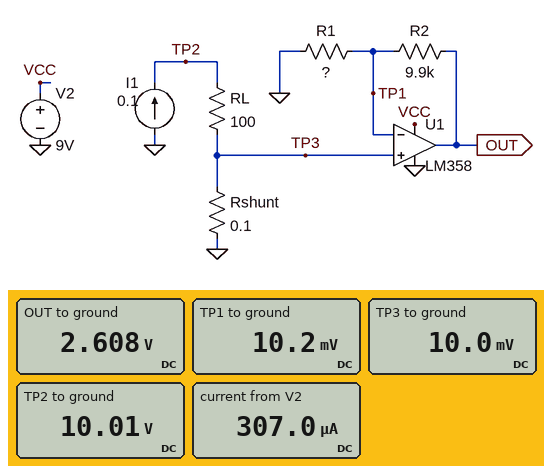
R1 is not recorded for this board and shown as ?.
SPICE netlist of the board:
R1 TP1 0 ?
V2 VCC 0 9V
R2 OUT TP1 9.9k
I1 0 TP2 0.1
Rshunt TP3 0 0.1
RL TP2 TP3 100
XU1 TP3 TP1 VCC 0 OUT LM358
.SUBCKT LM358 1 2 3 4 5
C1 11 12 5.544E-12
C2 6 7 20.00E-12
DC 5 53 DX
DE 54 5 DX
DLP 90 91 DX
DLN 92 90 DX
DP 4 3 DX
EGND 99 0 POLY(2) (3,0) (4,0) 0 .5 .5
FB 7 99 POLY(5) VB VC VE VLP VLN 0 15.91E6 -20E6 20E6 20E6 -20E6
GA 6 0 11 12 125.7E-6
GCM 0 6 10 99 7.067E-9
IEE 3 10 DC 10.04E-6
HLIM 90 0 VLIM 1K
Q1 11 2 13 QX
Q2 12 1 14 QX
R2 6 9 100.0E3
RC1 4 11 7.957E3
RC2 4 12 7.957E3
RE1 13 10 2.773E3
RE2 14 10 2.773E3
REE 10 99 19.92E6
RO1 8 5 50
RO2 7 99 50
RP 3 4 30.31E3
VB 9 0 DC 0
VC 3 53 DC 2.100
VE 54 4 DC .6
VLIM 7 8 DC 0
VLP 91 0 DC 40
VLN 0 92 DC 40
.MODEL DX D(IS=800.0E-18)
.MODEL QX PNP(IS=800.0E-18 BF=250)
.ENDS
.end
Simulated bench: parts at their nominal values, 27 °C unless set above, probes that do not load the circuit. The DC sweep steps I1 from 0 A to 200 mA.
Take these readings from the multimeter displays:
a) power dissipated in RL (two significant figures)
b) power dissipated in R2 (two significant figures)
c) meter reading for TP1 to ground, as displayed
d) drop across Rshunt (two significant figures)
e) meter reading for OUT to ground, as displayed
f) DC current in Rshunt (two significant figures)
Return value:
1.0 W
680 µW
10.2 mV
10 mV
2.608 V
100 mA
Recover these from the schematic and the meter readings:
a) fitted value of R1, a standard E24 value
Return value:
39 Ω
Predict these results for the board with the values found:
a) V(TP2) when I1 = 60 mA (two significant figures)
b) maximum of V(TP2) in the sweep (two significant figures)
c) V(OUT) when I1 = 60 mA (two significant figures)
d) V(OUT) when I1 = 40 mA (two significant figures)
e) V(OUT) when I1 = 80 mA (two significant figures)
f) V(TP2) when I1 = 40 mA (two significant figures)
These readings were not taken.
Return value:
6.0 V
20 V
1.6 V
1.1 V
2.1 V
4.0 V
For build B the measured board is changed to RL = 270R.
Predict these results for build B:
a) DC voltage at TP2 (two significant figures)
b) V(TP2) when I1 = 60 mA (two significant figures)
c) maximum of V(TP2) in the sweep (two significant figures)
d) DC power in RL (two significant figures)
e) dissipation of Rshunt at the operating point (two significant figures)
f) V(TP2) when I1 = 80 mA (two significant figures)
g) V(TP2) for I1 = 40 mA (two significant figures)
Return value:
27 V
16 V
54 V
2.7 W
1.0 mW
22 V
11 V
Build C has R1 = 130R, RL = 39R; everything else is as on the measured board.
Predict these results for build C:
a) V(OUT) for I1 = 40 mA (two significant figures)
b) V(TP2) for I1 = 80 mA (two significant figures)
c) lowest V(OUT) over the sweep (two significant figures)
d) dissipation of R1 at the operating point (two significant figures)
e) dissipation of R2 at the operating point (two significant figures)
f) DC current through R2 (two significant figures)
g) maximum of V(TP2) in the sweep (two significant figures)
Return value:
330 mV
3.1 V
110 mV
810 nW
62 µW
79 µA
7.8 V
